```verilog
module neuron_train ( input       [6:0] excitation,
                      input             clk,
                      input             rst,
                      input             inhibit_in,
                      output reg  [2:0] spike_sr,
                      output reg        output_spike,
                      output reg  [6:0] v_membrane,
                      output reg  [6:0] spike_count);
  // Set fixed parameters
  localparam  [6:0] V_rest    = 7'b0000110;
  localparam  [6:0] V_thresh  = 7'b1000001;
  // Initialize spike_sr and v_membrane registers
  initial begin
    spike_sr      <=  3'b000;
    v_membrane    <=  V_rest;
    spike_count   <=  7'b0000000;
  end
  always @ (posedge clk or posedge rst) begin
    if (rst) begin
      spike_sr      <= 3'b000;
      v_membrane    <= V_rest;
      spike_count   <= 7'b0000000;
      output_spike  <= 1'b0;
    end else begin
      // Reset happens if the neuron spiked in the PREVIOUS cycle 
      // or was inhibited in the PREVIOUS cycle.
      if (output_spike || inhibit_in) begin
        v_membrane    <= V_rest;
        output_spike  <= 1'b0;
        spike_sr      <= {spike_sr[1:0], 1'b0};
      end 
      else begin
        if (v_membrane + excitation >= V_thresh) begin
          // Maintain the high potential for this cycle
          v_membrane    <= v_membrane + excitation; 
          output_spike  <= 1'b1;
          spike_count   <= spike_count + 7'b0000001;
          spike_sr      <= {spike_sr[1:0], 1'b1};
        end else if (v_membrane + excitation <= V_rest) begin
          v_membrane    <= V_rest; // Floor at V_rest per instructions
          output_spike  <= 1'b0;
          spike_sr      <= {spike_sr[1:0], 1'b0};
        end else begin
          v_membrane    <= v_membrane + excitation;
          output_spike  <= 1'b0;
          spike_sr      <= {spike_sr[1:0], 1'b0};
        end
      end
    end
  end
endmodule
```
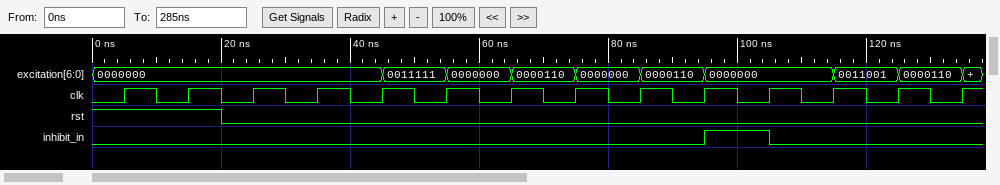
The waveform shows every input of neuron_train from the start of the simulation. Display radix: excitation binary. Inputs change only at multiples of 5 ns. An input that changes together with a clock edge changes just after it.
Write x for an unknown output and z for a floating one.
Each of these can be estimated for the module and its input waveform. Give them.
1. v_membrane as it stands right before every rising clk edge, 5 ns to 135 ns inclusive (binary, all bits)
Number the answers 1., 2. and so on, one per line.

1. 0000110, 0000110, 0000110, 0000110, 0000110, 0000110, 0100101, 0100101, 0101011, 0101011, 0110001, 0000110, 0000110, 0011111
